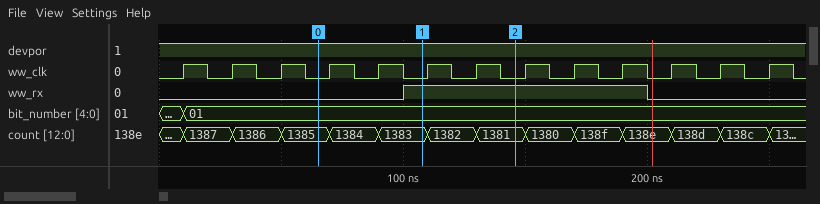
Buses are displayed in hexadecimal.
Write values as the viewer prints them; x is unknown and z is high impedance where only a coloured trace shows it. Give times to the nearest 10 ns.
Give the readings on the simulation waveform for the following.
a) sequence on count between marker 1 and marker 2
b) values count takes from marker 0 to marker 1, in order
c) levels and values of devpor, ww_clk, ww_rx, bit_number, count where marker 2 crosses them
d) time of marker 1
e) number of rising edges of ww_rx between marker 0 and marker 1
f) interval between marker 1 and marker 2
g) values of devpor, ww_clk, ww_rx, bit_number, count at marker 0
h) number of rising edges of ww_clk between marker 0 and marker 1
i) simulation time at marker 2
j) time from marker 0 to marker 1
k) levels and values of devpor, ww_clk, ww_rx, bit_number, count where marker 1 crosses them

1383, 1382, 1381
1385, 1384, 1383
devpor=1, ww_clk=0, ww_rx=1, bit_number=01, count=1381
110 ns
1
40 ns
devpor=1, ww_clk=0, ww_rx=0, bit_number=01, count=1385
2
150 ns
40 ns
devpor=1, ww_clk=0, ww_rx=1, bit_number=01, count=1383
